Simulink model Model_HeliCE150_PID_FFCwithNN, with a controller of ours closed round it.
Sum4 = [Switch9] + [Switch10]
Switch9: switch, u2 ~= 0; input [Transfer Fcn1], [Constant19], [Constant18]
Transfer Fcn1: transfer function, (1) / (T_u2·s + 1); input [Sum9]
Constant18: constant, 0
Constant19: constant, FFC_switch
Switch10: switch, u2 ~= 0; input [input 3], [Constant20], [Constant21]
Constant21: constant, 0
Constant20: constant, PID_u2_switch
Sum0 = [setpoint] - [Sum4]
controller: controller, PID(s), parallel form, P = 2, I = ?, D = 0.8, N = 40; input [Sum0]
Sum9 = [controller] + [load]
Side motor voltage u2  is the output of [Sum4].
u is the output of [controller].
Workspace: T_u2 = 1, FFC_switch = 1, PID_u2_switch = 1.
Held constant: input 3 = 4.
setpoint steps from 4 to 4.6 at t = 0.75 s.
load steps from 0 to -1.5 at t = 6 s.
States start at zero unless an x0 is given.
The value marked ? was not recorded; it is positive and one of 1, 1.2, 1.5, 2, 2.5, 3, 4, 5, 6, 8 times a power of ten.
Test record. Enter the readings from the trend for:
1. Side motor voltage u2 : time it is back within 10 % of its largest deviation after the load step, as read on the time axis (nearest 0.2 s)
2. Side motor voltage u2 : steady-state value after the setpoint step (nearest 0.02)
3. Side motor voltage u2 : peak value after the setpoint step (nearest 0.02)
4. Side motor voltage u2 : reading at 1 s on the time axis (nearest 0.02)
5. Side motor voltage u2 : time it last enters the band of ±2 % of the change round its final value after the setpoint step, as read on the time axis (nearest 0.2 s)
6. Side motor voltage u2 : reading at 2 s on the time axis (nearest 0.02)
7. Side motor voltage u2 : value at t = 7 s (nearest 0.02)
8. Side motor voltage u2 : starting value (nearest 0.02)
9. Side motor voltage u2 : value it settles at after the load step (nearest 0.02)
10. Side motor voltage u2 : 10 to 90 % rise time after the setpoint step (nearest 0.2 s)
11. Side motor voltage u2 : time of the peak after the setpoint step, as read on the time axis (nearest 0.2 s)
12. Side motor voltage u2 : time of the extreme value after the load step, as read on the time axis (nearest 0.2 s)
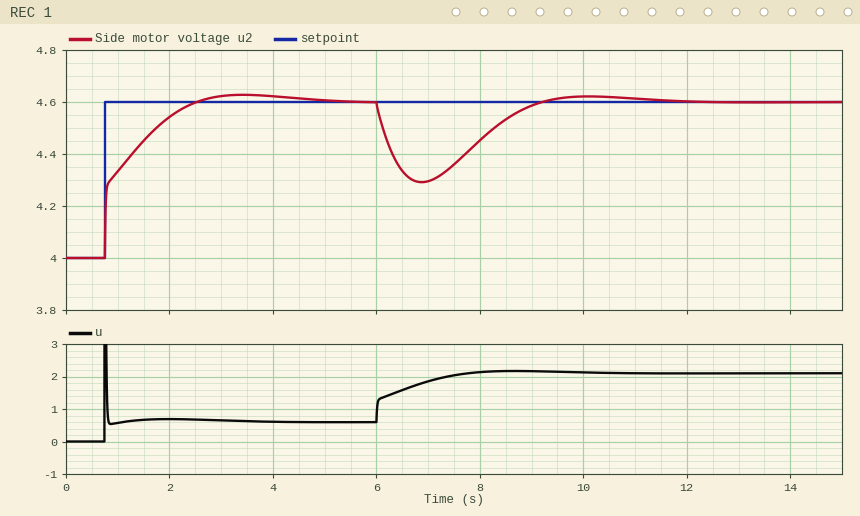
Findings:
8.8 s
4.60
4.62
4.34
4.6 s
4.54
4.30
4.00
4.60
1.2 s
3.4 s
6.8 s
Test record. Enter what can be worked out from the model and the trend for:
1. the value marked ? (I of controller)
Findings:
3
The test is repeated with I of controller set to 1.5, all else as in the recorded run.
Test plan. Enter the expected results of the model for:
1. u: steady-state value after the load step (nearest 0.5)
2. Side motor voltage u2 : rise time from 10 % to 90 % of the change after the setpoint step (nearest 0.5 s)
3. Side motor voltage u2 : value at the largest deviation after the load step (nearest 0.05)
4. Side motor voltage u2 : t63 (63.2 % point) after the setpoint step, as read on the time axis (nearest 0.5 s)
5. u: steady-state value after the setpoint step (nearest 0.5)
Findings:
2.0
2.0 s
4.25
1.5 s
0.5
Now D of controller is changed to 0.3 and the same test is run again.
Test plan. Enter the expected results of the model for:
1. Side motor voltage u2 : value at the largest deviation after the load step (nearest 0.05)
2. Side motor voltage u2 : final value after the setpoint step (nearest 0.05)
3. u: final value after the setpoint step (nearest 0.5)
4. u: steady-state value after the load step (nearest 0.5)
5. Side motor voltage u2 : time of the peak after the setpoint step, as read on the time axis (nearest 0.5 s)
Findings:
4.25
4.60
0.5
2.0
3.0 s
